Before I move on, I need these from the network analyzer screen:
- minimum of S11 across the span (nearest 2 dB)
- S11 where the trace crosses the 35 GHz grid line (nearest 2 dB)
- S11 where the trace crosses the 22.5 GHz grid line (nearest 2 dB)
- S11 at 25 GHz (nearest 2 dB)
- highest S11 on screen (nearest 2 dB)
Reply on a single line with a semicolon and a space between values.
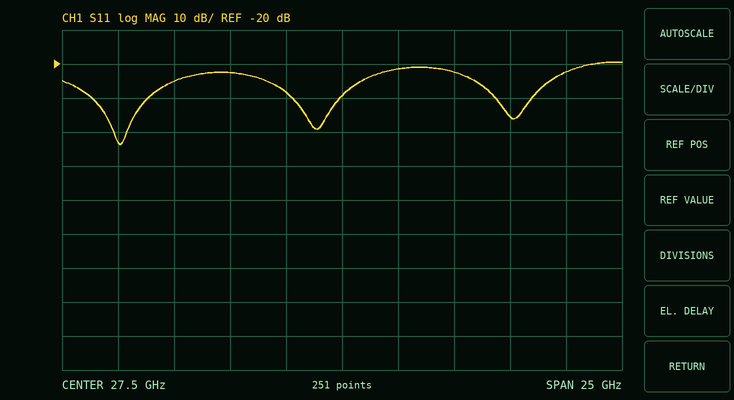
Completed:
-44 dB; -36 dB; -22 dB; -28 dB; -20 dB
